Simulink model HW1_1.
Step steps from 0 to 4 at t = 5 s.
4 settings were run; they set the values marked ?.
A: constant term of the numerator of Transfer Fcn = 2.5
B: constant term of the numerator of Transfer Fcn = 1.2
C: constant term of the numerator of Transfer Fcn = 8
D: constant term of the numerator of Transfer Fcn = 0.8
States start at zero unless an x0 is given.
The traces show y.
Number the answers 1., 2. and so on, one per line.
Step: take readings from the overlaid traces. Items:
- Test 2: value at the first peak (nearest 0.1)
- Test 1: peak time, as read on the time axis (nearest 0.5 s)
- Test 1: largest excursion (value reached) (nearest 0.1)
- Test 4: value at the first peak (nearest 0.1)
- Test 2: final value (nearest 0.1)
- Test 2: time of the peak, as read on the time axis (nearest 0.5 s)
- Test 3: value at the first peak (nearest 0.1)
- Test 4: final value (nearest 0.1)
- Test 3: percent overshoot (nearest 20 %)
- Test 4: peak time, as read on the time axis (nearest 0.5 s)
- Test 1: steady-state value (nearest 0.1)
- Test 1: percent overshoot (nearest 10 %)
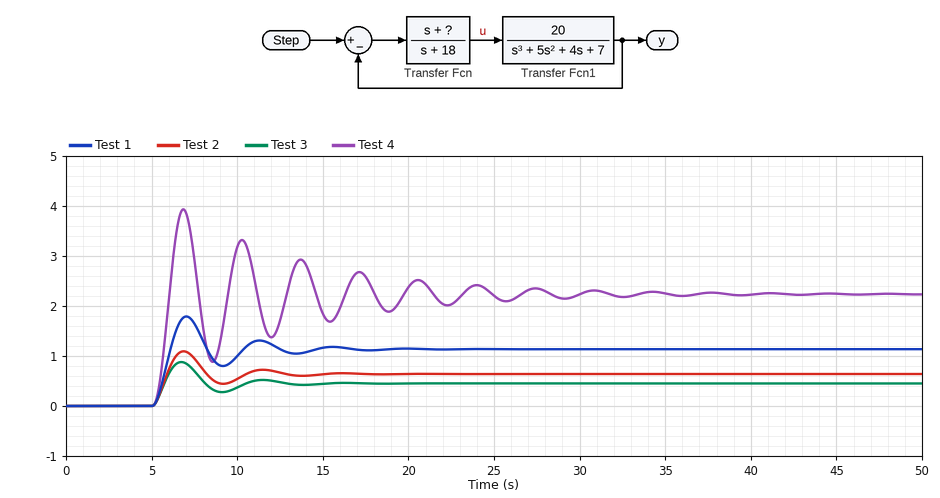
1. 1.1
2. 7.0 s
3. 1.8
4. 3.9
5. 0.6
6. 7.0 s
7. 0.9
8. 2.2
9. 100 %
10. 7.0 s
11. 1.1
12. 60 %
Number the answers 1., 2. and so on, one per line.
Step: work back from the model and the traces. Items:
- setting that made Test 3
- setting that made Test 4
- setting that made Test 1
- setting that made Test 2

1. D
2. C
3. A
4. B
